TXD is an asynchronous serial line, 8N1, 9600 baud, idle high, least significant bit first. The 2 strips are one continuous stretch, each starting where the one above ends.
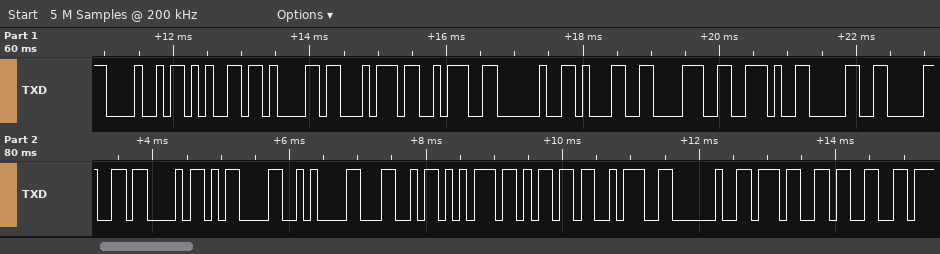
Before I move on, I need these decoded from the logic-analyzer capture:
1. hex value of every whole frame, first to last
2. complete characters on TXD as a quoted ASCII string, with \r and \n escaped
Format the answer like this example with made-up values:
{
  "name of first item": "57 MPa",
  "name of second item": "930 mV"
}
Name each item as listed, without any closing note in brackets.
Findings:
{
  "hex value of every whole frame, first to last": "48 65 61 74 3A 20 31 38 2E 30 30 43 0D 0A 4C 75 6D 3A 20 37 33",
  "complete characters on TXD as a quoted ASCII string, with \\r and \\n escaped": "\"Heat: 18.00C\\r\\nLum: 73\""
}
